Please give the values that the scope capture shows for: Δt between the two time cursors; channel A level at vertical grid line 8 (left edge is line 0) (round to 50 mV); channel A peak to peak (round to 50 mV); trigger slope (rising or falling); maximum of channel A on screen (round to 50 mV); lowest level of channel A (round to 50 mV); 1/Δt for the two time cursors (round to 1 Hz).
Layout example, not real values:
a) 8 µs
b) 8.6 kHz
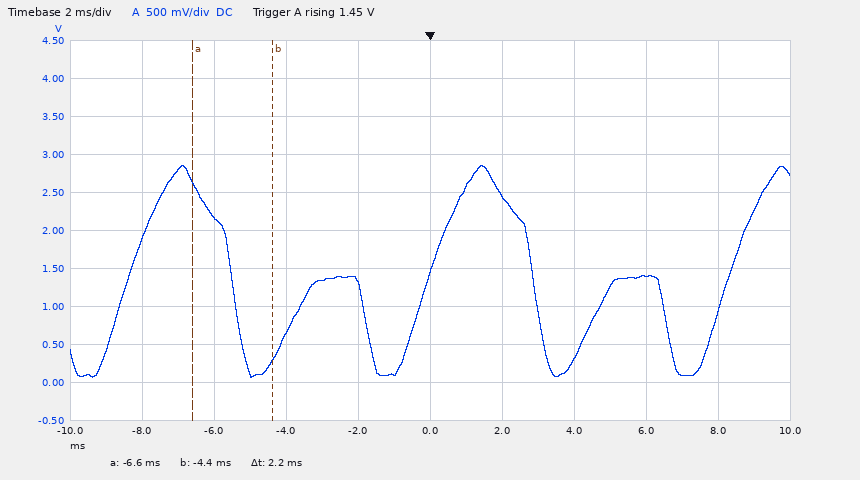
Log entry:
a) 2.2 ms
b) 1.40 V
c) 2.80 V
d) rising
e) 2.85 V
f) 50 mV
g) 455 Hz
